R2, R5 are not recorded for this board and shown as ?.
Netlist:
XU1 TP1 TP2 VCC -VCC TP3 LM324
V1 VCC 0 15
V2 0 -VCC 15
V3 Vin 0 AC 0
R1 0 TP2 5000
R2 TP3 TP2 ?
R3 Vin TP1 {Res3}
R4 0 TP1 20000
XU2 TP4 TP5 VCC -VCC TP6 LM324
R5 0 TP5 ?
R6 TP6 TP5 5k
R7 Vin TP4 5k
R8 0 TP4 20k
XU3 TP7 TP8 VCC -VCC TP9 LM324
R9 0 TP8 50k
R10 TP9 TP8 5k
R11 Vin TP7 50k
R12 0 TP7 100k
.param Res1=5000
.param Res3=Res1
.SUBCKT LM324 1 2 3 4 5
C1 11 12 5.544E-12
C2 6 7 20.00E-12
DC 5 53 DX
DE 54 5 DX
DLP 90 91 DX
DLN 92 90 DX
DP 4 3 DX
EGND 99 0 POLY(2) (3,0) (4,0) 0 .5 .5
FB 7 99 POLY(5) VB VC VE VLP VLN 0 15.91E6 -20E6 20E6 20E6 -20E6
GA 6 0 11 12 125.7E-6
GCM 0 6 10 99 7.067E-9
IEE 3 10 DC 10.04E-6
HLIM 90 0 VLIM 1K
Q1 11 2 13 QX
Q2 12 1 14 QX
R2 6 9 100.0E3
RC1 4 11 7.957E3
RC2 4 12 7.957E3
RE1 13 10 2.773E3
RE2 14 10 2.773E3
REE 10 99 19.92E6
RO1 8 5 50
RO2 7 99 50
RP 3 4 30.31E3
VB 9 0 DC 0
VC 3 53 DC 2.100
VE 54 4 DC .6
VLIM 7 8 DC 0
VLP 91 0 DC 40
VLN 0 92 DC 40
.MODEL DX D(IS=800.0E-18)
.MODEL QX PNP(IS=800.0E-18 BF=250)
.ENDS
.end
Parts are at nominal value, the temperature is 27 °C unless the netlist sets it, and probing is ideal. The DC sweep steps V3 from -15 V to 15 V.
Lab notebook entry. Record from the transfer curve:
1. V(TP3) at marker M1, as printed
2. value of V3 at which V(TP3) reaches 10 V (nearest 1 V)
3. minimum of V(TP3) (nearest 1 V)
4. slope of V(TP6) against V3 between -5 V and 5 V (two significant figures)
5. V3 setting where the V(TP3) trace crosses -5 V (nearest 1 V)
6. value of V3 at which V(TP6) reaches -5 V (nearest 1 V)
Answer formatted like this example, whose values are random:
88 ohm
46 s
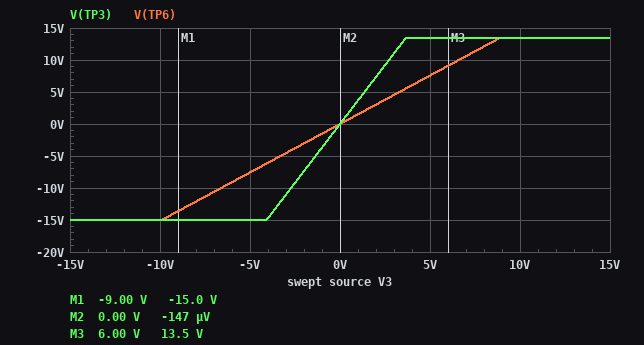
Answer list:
-15.0 V
3 V
-15 V
1.5 V/V
-1 V
-3 V
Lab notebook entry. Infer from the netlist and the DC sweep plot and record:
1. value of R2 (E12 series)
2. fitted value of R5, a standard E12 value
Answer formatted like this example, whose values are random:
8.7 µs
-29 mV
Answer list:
18 kΩ
5.6 kΩ
